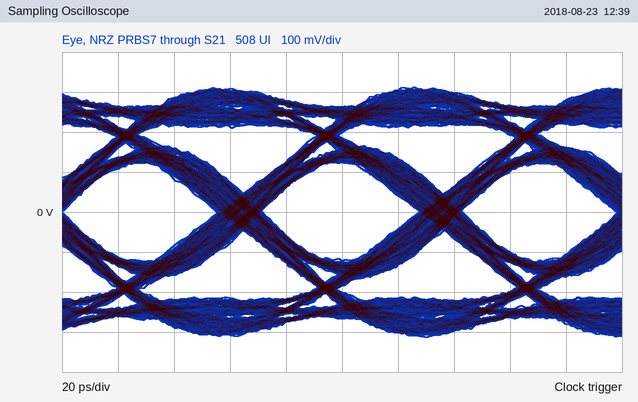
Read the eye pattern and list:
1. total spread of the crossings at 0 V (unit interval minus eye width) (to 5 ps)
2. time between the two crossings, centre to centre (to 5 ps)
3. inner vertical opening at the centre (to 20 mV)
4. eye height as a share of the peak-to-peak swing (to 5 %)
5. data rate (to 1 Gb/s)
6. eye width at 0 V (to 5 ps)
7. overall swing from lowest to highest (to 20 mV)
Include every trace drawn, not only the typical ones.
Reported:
15 ps
70 ps
240 mV
40 %
14 Gb/s
55 ps
620 mV
